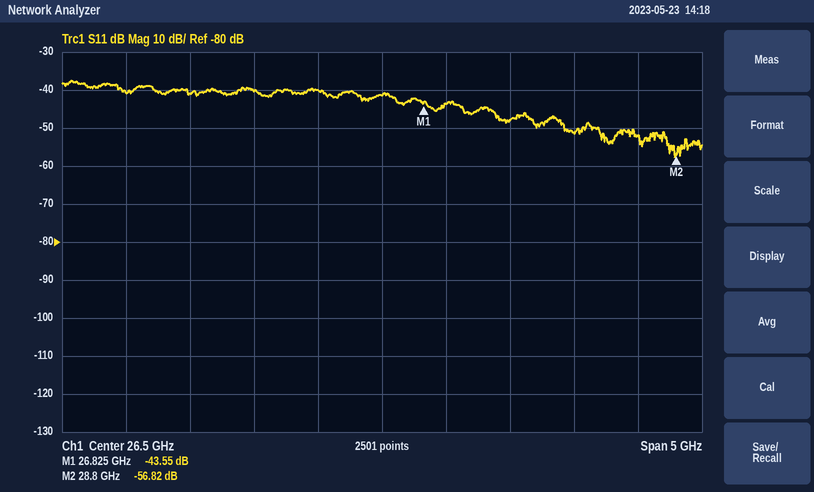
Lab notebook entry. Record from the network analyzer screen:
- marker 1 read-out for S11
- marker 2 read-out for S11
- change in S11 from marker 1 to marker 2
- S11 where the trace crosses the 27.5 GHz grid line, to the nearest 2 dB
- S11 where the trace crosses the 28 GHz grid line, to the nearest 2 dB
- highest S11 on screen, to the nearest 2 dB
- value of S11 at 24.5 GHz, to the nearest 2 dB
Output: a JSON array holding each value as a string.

["-43.55 dB", "-56.82 dB", "-13.27 dB", "-48 dB", "-52 dB", "-38 dB", "-40 dB"]
